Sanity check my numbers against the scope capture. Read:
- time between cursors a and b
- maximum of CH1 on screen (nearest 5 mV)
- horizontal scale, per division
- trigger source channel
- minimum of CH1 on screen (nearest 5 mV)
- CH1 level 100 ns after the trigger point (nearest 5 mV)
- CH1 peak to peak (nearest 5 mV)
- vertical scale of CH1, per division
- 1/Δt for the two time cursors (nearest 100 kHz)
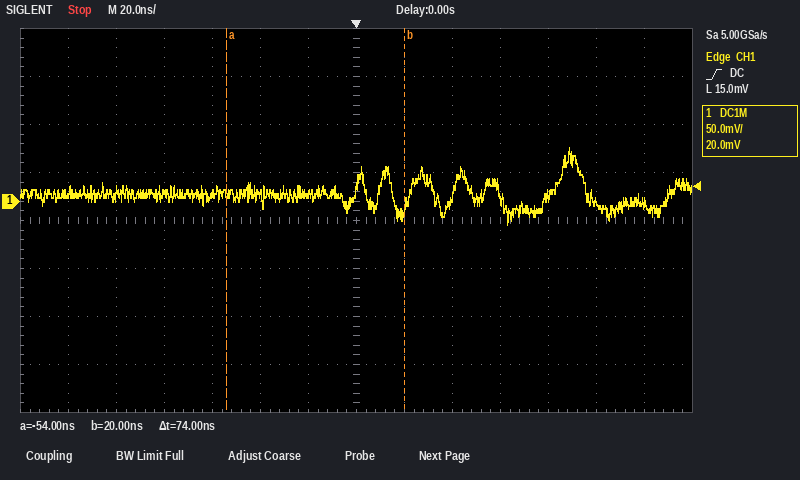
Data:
74 ns
55 mV
20 ns
CH1
-25 mV
0 mV
80 mV
50 mV
13.5 MHz
